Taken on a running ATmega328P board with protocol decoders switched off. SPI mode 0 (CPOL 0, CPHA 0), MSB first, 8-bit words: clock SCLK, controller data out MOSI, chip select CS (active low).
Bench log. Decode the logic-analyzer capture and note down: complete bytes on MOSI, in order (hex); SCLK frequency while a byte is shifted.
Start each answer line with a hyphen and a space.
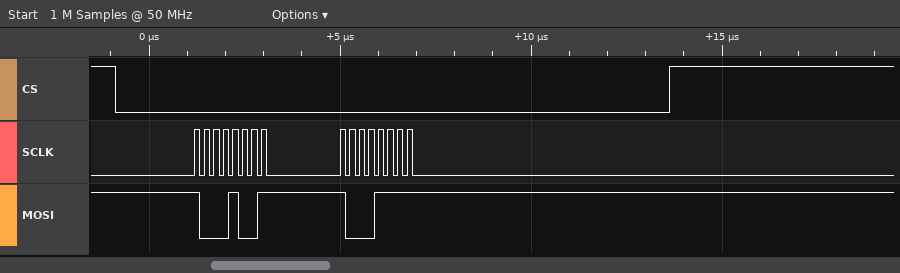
- 89 8F
- 4 MHz
